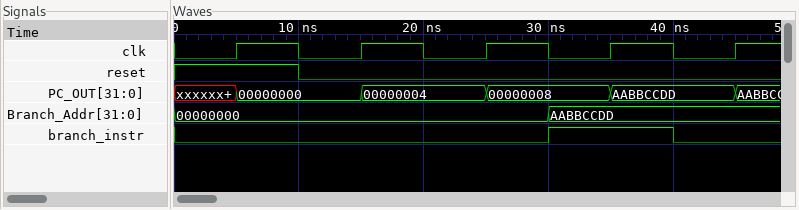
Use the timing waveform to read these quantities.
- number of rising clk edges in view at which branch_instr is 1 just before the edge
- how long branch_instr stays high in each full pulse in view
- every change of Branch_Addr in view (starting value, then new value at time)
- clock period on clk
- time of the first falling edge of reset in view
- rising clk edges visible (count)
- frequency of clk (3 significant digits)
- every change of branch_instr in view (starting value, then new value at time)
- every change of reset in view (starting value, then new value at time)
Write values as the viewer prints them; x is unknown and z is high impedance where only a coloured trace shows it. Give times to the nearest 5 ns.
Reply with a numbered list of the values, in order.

1. 1
2. 10 ns
3. 00000000, AABBCCDD at 30 ns
4. 10 ns
5. 10 ns
6. 5
7. 100 MHz
8. 0, 1 at 30 ns, 0 at 40 ns
9. 1, 0 at 10 ns
